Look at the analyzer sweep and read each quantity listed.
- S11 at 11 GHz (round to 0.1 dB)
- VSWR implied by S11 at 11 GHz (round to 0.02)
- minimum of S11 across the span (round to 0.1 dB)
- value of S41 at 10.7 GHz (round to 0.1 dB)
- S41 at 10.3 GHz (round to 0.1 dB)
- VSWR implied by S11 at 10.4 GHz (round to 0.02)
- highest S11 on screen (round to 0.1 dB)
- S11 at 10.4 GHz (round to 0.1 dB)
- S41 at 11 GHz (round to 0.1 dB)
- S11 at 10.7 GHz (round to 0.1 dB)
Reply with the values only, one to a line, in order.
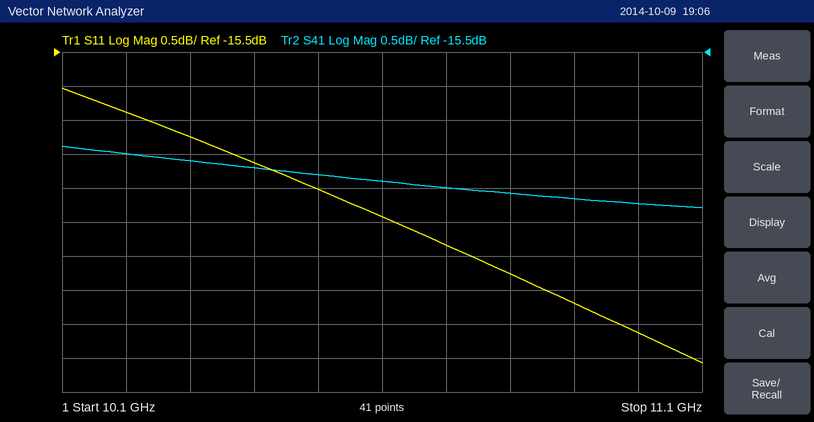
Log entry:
-19.6 dB
1.24
-20.1 dB
-17.5 dB
-17.1 dB
1.32
-16.0 dB
-17.1 dB
-17.7 dB
-18.3 dB
